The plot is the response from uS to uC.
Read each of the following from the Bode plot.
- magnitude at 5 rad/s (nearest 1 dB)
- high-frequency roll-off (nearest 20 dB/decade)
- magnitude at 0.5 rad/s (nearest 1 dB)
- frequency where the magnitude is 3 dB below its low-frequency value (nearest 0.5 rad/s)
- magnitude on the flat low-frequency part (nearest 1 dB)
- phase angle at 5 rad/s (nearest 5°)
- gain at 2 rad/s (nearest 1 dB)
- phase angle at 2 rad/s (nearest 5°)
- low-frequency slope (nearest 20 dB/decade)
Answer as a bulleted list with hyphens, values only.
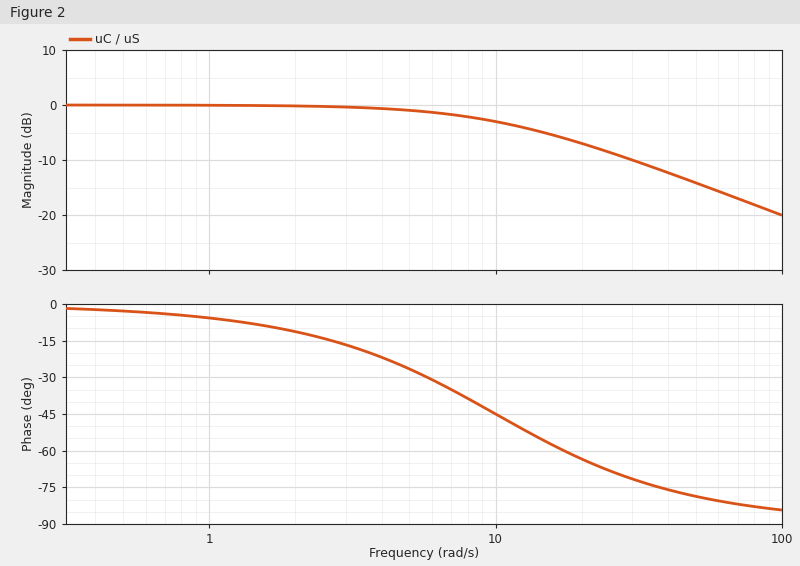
- -1 dB
- -20 dB/decade
- 0 dB
- 10.0 rad/s
- 0 dB
- -25°
- 0 dB
- -10°
- 0 dB/decade
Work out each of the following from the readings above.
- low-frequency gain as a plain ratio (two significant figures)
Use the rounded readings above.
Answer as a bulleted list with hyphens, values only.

- 1.0
